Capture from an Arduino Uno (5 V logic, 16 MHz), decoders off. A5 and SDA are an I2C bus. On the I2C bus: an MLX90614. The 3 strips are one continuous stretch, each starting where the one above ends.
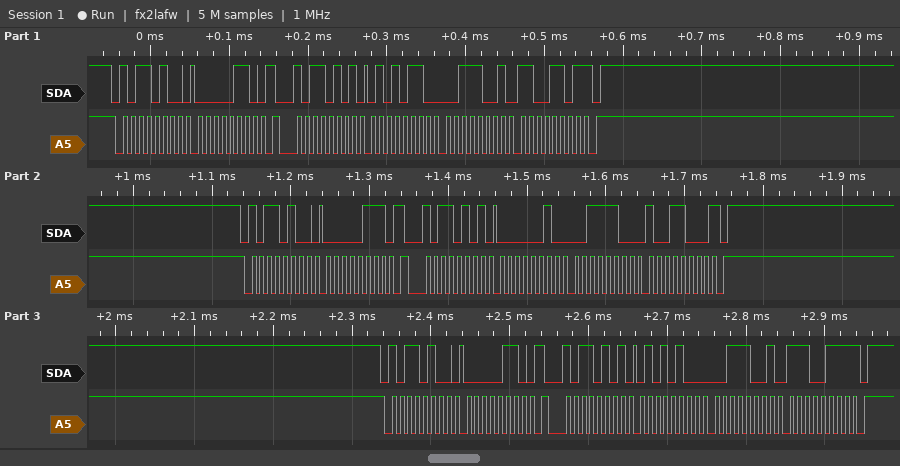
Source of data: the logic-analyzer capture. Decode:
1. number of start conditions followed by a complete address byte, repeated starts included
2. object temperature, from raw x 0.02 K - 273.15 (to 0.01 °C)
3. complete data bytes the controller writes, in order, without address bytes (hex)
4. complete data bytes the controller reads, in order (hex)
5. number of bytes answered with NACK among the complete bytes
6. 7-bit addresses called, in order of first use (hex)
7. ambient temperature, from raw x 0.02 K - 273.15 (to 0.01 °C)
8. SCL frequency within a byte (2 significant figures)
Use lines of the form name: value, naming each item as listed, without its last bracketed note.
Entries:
number of start conditions followed by a complete address byte, repeated starts included: 6
object temperature, from raw x 0.02 K - 273.15: 34.09 °C
complete data bytes the controller writes, in order, without address bytes: 06 07 06
complete data bytes the controller reads, in order: 56 39 CD 02 3C 98 54 39 E7
number of bytes answered with NACK among the complete bytes: 3
7-bit addresses called, in order of first use: 0x5A
ambient temperature, from raw x 0.02 K - 273.15: 20.41 °C
SCL frequency within a byte: 100 kHz
